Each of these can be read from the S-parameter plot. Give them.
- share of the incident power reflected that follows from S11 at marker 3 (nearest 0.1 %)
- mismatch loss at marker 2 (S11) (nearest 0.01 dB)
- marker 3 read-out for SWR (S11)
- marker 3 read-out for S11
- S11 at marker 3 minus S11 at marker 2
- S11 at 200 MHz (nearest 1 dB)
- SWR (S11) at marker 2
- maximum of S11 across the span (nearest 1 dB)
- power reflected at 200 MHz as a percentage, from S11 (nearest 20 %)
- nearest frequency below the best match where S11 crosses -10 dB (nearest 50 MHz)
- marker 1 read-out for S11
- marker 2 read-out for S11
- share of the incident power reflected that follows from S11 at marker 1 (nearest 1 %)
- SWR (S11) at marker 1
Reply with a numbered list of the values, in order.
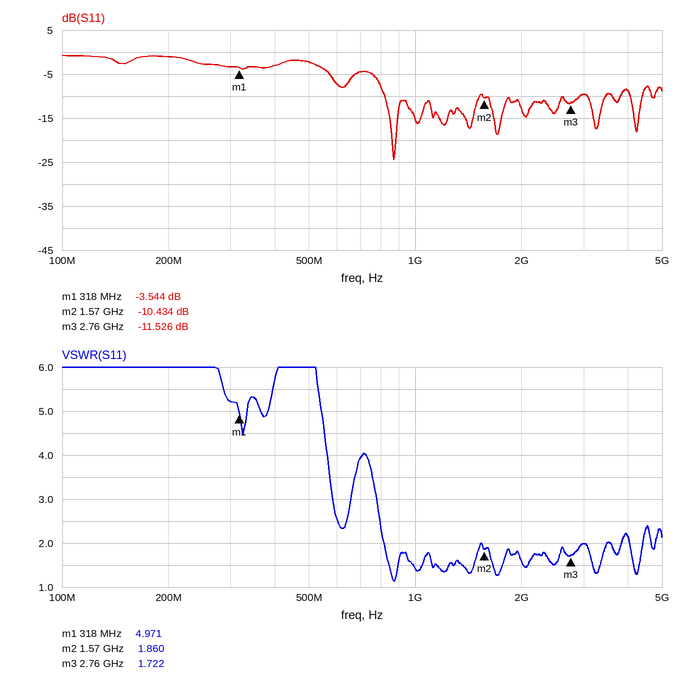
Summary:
1. 7.0 %
2. 0.41 dB
3. 1.722
4. -11.526 dB
5. -1.092 dB
6. -1 dB
7. 1.860
8. -1 dB
9. 80 %
10. 800 MHz
11. -3.544 dB
12. -10.434 dB
13. 44 %
14. 4.971
